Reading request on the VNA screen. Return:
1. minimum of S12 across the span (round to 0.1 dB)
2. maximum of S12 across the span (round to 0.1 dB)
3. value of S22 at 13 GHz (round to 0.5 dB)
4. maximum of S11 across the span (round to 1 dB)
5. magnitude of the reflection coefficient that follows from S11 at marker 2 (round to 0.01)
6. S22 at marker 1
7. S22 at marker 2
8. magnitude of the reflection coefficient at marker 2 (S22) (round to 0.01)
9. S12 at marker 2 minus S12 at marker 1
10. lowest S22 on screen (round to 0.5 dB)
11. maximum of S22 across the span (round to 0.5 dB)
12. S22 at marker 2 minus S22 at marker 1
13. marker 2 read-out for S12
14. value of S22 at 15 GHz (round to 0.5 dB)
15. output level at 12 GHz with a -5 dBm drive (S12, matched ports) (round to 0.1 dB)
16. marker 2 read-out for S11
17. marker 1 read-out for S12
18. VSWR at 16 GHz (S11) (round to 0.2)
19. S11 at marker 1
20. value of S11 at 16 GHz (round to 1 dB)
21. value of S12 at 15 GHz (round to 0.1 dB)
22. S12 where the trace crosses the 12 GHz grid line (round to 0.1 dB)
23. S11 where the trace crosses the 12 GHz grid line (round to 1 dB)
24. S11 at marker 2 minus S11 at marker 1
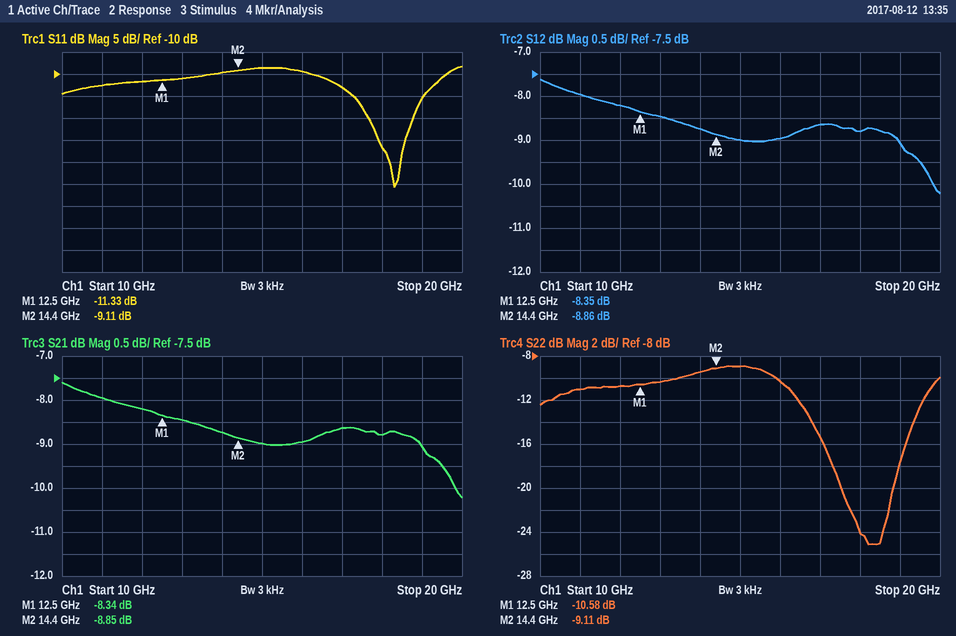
-10.2 dB
-7.6 dB
-10.5 dB
-8 dB
0.35
-10.58 dB
-9.11 dB
0.35
-0.51 dB
-25.0 dB
-9.0 dB
1.47 dB
-8.86 dB
-9.0 dB
-13.2 dBm
-9.11 dB
-8.35 dB
2.0
-11.33 dB
-9 dB
-9.0 dB
-8.2 dB
-12 dB
2.22 dB
